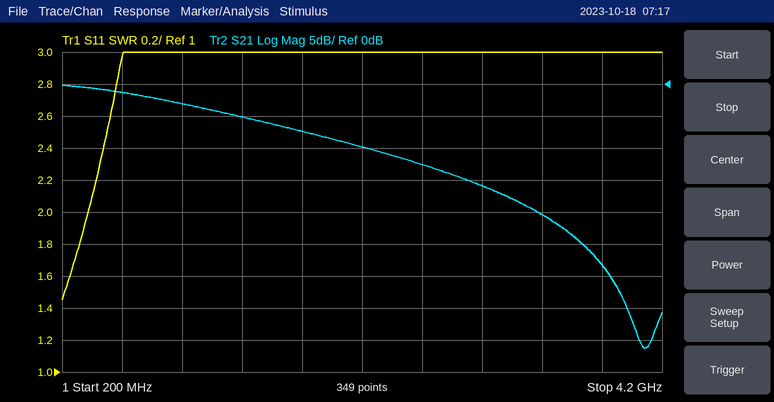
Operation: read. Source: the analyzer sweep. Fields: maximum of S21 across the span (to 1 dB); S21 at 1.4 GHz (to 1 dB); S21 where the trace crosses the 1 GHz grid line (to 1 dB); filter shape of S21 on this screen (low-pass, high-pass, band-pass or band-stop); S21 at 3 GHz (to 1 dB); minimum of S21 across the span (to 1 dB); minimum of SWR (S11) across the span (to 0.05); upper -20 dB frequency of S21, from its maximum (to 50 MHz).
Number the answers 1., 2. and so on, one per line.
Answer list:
1. 0 dB
2. -5 dB
3. -3 dB
4. low-pass
5. -16 dB
6. -41 dB
7. 1.45
8. 3.40 GHz
